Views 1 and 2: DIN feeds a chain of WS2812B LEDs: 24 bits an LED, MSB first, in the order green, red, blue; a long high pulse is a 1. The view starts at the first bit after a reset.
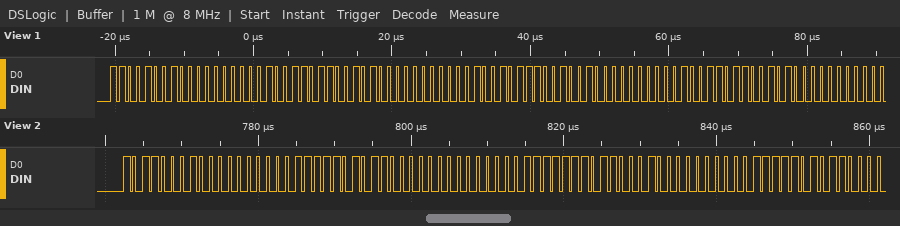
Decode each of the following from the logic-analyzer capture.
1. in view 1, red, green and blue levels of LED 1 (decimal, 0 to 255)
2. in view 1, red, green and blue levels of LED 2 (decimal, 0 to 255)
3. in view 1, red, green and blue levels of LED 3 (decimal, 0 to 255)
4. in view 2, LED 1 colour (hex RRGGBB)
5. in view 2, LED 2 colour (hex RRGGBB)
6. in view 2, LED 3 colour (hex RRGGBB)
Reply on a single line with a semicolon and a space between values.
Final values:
0, 201, 38; 0, 202, 37; 0, 201, 38; #00B13E; #00B03F; #00B13E
